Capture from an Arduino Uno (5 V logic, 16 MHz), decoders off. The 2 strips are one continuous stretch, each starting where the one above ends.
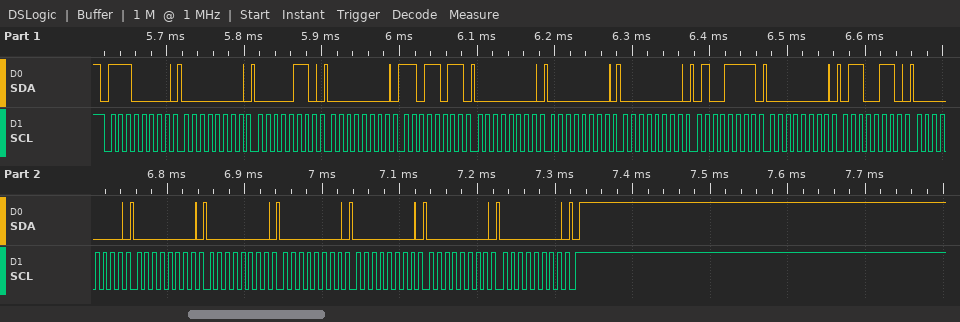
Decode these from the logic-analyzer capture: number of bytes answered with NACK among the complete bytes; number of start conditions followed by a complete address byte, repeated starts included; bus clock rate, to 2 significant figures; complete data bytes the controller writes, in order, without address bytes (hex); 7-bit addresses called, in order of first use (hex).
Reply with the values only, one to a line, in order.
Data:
0
1
100 kHz
00 06 00 DB 00 00 00 4F 00 66 00 00 00 00 00 00 00
0x70
